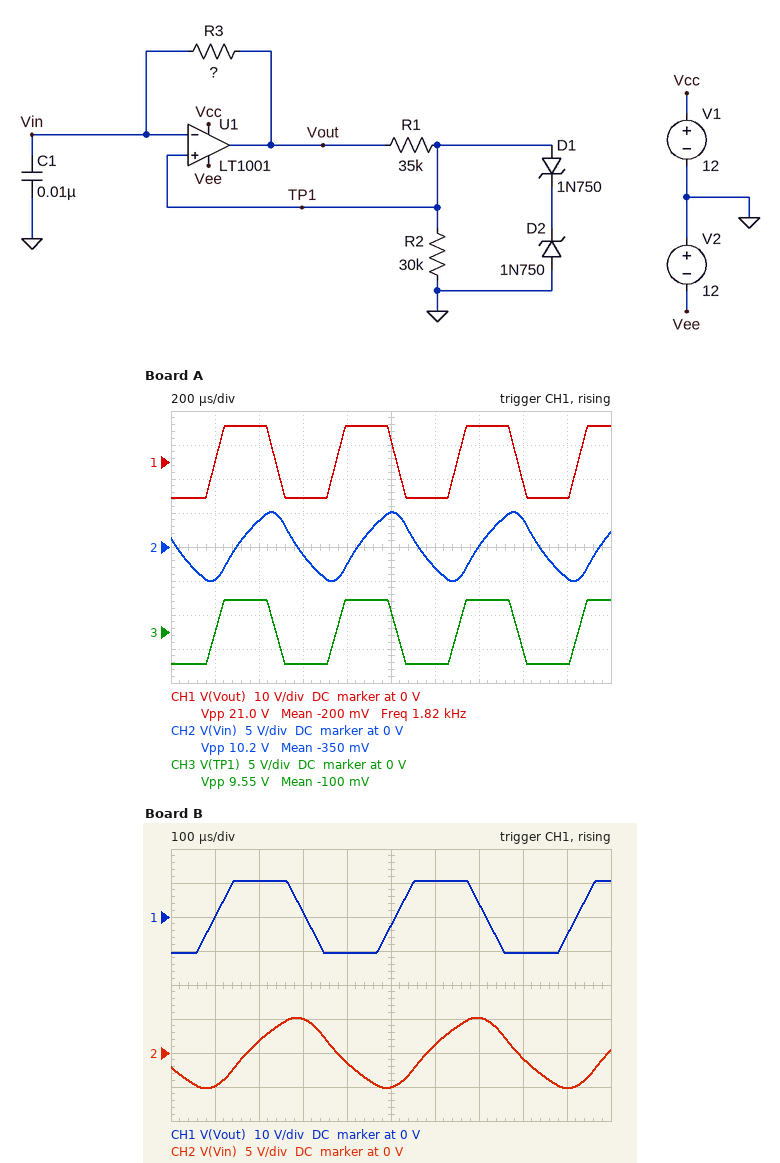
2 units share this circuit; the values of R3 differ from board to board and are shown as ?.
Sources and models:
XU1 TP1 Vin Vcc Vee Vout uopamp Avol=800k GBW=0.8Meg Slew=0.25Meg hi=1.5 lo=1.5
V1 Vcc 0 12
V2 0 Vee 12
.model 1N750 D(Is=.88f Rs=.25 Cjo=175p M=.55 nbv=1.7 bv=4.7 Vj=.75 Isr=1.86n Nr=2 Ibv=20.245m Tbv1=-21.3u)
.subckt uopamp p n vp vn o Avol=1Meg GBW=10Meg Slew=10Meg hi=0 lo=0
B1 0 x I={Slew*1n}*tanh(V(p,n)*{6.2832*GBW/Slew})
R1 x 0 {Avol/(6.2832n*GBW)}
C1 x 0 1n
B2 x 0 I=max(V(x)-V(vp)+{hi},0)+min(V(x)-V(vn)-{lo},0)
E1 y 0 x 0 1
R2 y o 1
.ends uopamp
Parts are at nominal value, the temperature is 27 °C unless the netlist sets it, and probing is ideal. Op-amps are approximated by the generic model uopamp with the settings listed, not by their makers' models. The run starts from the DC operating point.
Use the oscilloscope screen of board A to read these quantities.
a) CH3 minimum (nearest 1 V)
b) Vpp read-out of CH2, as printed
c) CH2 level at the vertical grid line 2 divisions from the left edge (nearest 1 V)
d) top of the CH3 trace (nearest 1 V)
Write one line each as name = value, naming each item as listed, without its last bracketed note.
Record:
CH3 minimum = -5 V
Vpp read-out of CH2, as printed = 10.2 V
CH2 level at the vertical grid line 2 divisions from the left edge = 4 V
top of the CH3 trace = 5 V
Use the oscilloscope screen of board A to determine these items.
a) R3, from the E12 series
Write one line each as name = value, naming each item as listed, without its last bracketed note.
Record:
R3, from the E12 series = 22 kΩ
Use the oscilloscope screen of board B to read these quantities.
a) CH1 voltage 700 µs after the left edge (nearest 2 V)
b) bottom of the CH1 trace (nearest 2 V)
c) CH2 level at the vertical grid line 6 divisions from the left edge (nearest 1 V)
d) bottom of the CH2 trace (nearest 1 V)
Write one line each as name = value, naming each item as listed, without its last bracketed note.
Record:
CH1 voltage 700 µs after the left edge = 4 V
bottom of the CH1 trace = -10 V
CH2 level at the vertical grid line 6 divisions from the left edge = 1 V
bottom of the CH2 trace = -5 V
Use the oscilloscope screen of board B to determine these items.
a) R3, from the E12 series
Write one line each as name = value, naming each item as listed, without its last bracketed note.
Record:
R3, from the E12 series = 15 kΩ
